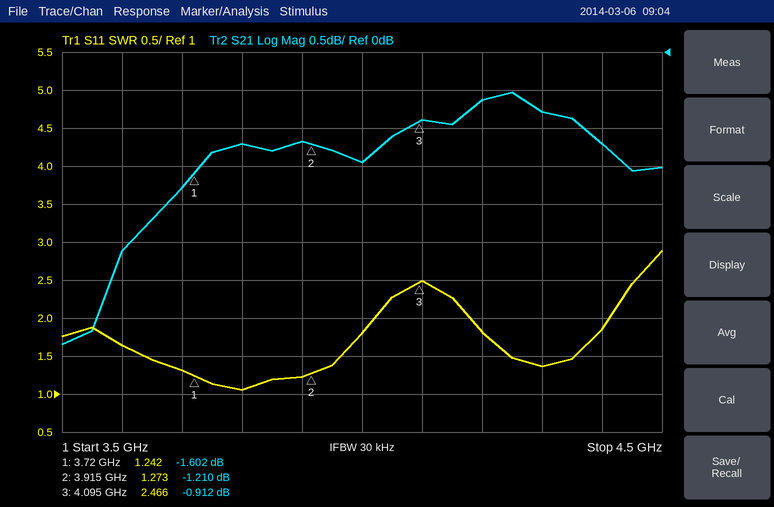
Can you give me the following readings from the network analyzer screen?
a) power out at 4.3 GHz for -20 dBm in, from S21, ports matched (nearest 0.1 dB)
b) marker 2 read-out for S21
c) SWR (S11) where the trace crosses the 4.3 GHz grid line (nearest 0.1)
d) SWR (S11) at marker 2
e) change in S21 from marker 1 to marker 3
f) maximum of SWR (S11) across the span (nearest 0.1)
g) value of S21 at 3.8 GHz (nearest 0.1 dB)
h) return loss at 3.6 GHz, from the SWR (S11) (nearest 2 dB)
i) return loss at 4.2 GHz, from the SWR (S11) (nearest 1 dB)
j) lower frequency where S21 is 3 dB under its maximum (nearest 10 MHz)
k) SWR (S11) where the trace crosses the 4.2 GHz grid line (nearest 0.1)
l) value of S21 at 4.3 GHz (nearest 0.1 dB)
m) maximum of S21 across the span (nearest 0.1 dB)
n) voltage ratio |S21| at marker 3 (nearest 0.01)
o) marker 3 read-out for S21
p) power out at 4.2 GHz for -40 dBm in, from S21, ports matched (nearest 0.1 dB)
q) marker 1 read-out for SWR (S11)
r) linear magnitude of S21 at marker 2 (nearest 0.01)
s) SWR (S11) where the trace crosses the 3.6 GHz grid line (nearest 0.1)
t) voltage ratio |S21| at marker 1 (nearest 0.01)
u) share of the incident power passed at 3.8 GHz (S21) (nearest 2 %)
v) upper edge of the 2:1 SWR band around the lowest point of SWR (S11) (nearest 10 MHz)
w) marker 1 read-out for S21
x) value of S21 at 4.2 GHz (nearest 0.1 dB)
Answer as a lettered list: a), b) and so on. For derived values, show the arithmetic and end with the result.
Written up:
a) -20 dBm + (-0.8 dB) = -20.8 dBm
b) -1.210 dB
c) 1.4
d) 1.273
e) -0.912 − (-1.602) = 0.690 dB
f) 2.9
g) -1.2 dB
h) −20 log10((1.6 − 1)/(1.6 + 1)) ≈ 12.7 dB, so 12 dB to the nearest 2 dB
i) −20 log10((1.8 − 1)/(1.8 + 1)) ≈ 11 dB
j) 3.56 GHz
k) 1.8
l) -0.8 dB
m) -0.5 dB
n) 10^(-0.912/20) ≈ 0.90
o) -0.912 dB
p) -40 dBm + (-0.6 dB) = -40.6 dBm
q) 1.242
r) 10^(-1.21/20) ≈ 0.87
s) 1.6
t) 10^(-1.602/20) ≈ 0.83
u) 10^(-1.2/10) ≈ 76 %
v) 4.02 GHz
w) -1.602 dB
x) -0.6 dB
